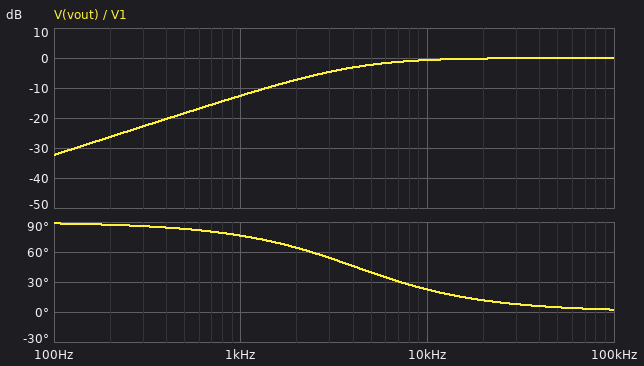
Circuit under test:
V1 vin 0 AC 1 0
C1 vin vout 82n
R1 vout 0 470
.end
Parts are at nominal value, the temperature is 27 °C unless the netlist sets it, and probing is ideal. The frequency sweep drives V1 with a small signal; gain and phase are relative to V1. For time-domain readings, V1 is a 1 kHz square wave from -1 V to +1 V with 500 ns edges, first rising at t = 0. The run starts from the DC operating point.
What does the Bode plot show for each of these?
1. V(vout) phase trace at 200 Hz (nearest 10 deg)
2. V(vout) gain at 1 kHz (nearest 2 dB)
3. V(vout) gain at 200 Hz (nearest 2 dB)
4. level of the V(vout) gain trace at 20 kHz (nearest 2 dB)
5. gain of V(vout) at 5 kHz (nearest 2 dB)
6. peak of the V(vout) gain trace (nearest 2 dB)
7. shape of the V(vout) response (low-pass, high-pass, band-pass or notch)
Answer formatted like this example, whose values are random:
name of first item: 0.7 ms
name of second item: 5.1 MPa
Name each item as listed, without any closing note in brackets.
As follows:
V(vout) phase trace at 200 Hz: 90 deg
V(vout) gain at 1 kHz: -12 dB
V(vout) gain at 200 Hz: -26 dB
level of the V(vout) gain trace at 20 kHz: 0 dB
gain of V(vout) at 5 kHz: -2 dB
peak of the V(vout) gain trace: 0 dB
shape of the V(vout) response: high-pass
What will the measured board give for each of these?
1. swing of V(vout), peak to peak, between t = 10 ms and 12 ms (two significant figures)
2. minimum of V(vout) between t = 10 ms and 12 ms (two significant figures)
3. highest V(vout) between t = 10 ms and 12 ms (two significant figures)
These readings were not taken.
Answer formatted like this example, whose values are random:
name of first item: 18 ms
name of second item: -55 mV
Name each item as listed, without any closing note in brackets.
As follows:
swing of V(vout), peak to peak, between t = 10 ms and 12 ms: 4.0 V
minimum of V(vout) between t = 10 ms and 12 ms: -2.0 V
highest V(vout) between t = 10 ms and 12 ms: 2.0 V
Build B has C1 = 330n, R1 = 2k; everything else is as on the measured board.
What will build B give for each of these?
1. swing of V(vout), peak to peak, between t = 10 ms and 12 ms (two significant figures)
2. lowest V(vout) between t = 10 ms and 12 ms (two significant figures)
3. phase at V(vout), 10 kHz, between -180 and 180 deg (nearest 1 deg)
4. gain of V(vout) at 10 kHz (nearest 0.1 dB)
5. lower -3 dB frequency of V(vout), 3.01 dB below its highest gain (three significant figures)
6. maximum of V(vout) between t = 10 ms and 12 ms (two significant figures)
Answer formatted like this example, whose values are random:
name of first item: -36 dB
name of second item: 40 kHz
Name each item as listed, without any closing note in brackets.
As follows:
swing of V(vout), peak to peak, between t = 10 ms and 12 ms: 2.7 V
lowest V(vout) between t = 10 ms and 12 ms: -1.4 V
phase at V(vout), 10 kHz, between -180 and 180 deg: 1 deg
gain of V(vout) at 10 kHz: 0 dB
lower -3 dB frequency of V(vout), 3.01 dB below its highest gain: 241 Hz
maximum of V(vout) between t = 10 ms and 12 ms: 1.4 V
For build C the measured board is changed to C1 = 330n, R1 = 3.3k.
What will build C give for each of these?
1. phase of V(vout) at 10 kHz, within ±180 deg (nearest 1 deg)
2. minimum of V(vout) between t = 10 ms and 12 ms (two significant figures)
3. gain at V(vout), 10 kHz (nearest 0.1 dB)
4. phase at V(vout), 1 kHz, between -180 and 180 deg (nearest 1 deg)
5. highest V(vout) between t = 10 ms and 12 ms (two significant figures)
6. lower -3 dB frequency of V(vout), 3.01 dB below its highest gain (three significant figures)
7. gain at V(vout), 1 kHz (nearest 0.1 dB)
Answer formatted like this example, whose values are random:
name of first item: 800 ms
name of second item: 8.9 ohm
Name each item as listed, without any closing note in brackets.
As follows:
phase of V(vout) at 10 kHz, within ±180 deg: 1 deg
minimum of V(vout) between t = 10 ms and 12 ms: -1.2 V
gain at V(vout), 10 kHz: 0 dB
phase at V(vout), 1 kHz, between -180 and 180 deg: 8 deg
highest V(vout) between t = 10 ms and 12 ms: 1.2 V
lower -3 dB frequency of V(vout), 3.01 dB below its highest gain: 146 Hz
gain at V(vout), 1 kHz: -0.1 dB
